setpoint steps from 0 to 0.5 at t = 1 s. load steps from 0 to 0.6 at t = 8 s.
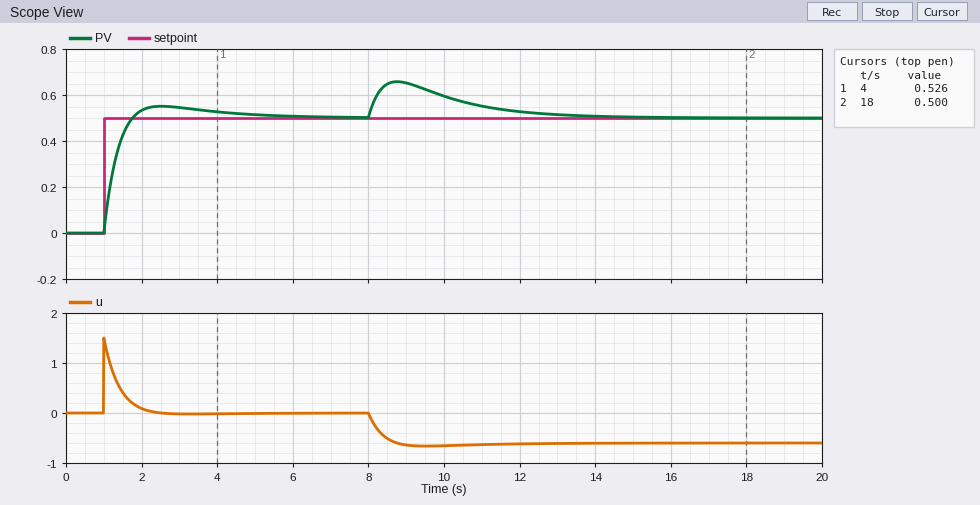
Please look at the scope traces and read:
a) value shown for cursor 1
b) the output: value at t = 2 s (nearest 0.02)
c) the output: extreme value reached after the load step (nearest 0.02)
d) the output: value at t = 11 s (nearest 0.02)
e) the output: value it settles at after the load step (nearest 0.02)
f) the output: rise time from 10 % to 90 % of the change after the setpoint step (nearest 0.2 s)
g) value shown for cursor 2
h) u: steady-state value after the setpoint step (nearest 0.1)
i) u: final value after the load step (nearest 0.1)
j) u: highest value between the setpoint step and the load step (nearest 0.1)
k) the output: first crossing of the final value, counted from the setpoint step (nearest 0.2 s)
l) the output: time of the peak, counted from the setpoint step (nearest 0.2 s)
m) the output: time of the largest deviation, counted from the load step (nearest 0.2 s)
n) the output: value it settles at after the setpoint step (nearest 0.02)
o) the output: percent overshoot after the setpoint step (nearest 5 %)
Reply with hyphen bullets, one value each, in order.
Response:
- 0.526
- 0.54
- 0.66
- 0.56
- 0.50
- 0.6 s
- 0.500
- 0.0
- -0.6
- 1.5
- 0.8 s
- 1.6 s
- 0.8 s
- 0.50
- 10 %
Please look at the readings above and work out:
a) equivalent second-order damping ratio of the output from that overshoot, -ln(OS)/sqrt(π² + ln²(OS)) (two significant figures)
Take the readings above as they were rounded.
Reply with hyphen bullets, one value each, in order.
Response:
- 0.59
